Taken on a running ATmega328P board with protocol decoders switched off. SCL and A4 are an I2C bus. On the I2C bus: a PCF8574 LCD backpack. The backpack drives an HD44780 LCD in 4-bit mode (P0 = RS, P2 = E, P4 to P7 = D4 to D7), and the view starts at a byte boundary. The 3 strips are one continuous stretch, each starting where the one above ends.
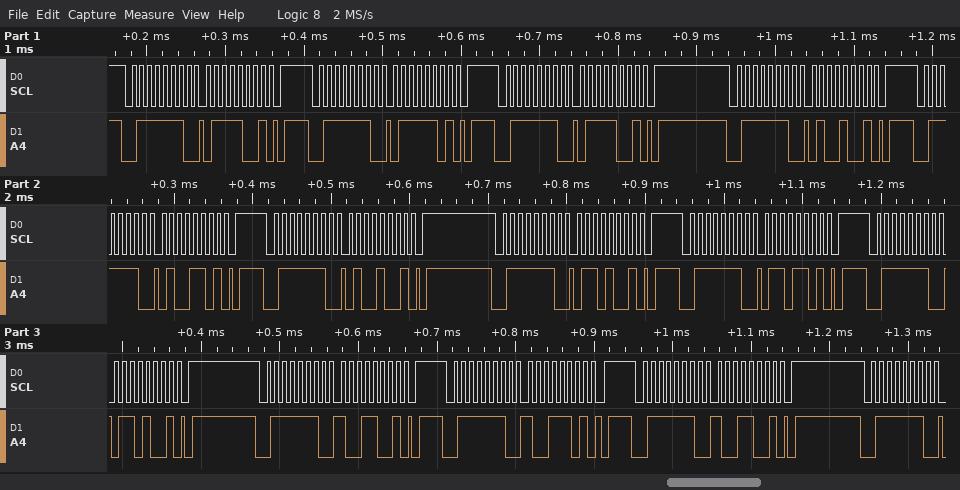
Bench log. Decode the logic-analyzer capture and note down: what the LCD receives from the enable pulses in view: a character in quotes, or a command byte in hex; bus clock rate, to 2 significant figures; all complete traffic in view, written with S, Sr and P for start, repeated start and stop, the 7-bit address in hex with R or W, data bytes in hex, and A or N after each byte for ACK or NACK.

't' 'i'
100 kHz
S 3FW A 79 A P S 3FW A 7D A P S 3FW A 79 A P S 3FW A 49 A P S 3FW A 4D A P S 3FW A 49 A P S 3FW A 69 A P S 3FW A 6D A P S 3FW A 69 A P S 3FW A 99 A P S 3FW A 9D A P S 3FW A 99 A P S 3FW A
